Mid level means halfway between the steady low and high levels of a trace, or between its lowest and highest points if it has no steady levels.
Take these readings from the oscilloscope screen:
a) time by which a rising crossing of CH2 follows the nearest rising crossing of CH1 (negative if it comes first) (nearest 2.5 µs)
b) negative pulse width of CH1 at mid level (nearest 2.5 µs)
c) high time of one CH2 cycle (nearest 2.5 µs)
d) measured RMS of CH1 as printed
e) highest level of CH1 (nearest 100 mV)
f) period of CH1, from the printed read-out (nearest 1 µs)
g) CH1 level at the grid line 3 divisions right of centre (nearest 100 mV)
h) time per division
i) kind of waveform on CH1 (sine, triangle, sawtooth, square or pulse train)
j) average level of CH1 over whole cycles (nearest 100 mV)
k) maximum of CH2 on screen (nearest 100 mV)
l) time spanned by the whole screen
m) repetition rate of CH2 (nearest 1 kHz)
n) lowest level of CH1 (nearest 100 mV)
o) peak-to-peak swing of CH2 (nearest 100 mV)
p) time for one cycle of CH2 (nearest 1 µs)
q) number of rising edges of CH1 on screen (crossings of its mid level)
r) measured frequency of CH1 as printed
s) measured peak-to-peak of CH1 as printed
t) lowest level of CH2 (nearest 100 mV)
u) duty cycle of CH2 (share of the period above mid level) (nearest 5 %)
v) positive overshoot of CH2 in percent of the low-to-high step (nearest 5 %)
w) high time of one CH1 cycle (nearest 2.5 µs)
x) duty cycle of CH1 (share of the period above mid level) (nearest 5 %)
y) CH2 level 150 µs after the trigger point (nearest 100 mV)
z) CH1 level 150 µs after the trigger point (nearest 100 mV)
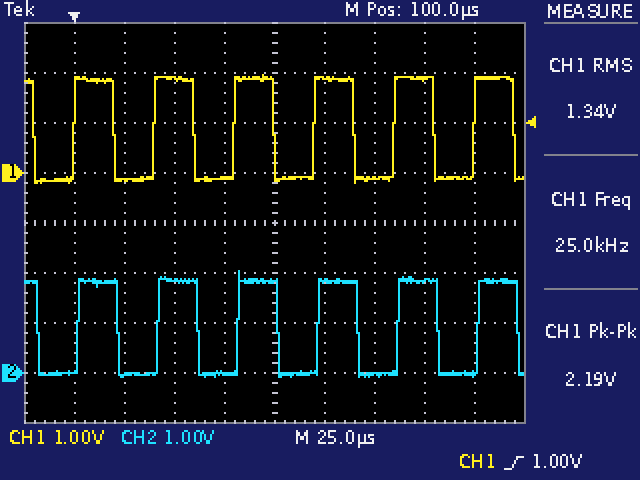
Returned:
+2.5 µs
20.0 µs
20.0 µs
1.34 V
2.0 V
40 µs
1.9 V
25 µs
square
900 mV
2.0 V
250 µs
25 kHz
-200 mV
2.1 V
40 µs
6
25.0 kHz
2.19 V
-100 mV
50 %
10 %
20.0 µs
50 %
0.0 V
-100 mV
